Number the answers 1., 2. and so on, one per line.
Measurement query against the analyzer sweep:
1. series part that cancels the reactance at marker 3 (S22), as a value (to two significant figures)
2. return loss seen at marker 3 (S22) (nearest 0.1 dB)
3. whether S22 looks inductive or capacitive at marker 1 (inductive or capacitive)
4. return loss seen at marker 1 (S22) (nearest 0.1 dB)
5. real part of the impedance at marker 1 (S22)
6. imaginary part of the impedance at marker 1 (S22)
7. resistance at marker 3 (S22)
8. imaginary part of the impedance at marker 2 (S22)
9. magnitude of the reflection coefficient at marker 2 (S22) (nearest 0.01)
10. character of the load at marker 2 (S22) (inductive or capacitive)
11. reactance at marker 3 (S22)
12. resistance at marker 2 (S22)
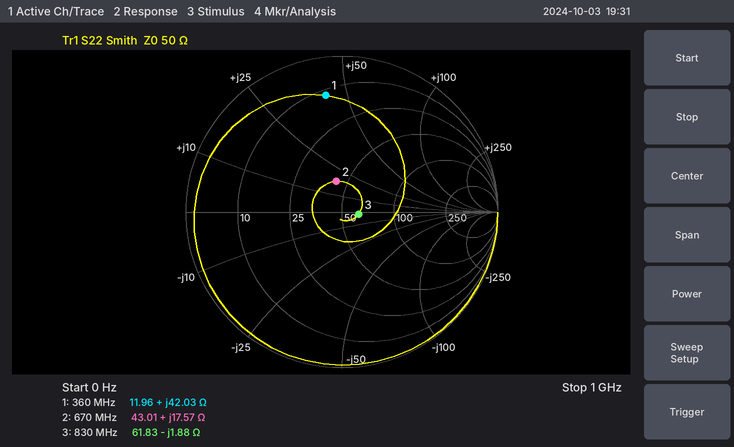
1. 360 pH
2. 19.4 dB
3. inductive
4. 2.4 dB
5. 11.96 Ω
6. +42.03 Ω
7. 61.83 Ω
8. +17.57 Ω
9. 0.20
10. inductive
11. -1.88 Ω
12. 43.01 Ω
